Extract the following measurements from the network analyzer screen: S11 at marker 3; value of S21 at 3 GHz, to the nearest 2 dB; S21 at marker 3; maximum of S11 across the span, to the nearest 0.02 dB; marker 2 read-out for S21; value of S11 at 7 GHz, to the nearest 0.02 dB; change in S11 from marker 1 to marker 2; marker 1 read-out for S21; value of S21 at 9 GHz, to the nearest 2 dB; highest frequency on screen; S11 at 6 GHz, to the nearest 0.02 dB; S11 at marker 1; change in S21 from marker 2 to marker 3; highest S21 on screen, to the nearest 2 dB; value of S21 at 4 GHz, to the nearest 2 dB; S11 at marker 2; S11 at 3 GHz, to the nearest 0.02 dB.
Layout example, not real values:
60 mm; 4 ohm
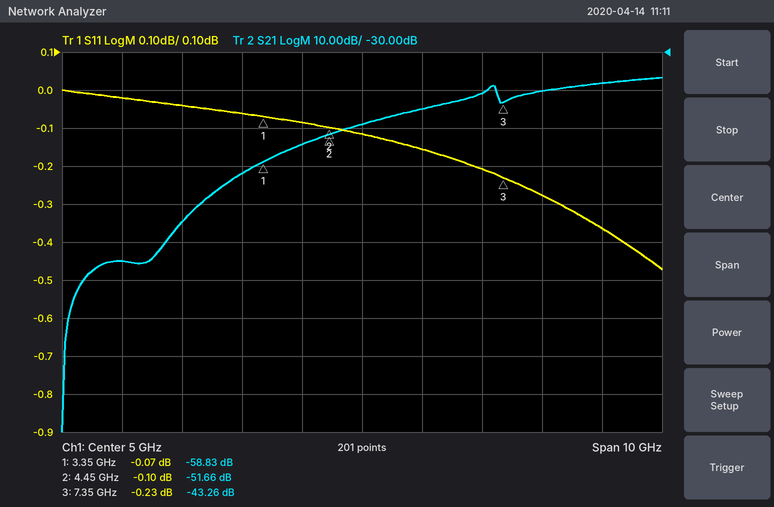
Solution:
-0.23 dB; -62 dB; -43.26 dB; 0.00 dB; -51.66 dB; -0.20 dB; -0.03 dB; -58.83 dB; -38 dB; 10 GHz; -0.16 dB; -0.07 dB; 8.40 dB; -36 dB; -54 dB; -0.10 dB; -0.06 dB
